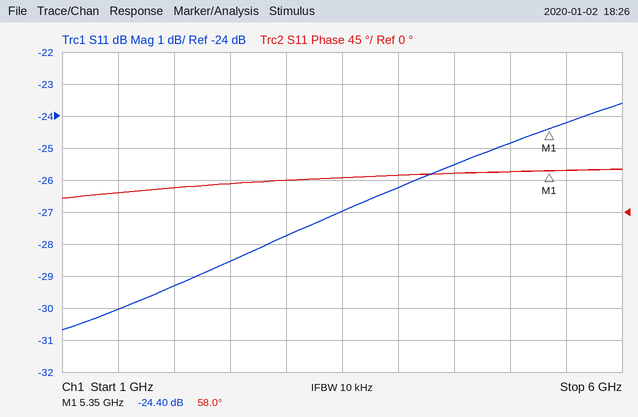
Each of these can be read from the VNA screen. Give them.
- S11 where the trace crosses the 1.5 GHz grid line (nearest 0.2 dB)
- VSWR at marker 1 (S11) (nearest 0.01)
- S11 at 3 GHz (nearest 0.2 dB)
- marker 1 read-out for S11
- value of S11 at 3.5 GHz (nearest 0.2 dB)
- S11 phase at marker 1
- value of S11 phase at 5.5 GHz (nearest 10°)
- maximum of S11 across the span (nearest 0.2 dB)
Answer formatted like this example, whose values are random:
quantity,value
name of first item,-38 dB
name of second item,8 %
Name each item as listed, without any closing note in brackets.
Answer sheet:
quantity,value
S11 where the trace crosses the 1.5 GHz grid line,-30.0 dB
VSWR at marker 1 (S11),1.13
S11 at 3 GHz,-27.8 dB
marker 1 read-out for S11,-24.40 dB
value of S11 at 3.5 GHz,-27.0 dB
S11 phase at marker 1,58.0°
value of S11 phase at 5.5 GHz,60°
maximum of S11 across the span,-23.6 dB
